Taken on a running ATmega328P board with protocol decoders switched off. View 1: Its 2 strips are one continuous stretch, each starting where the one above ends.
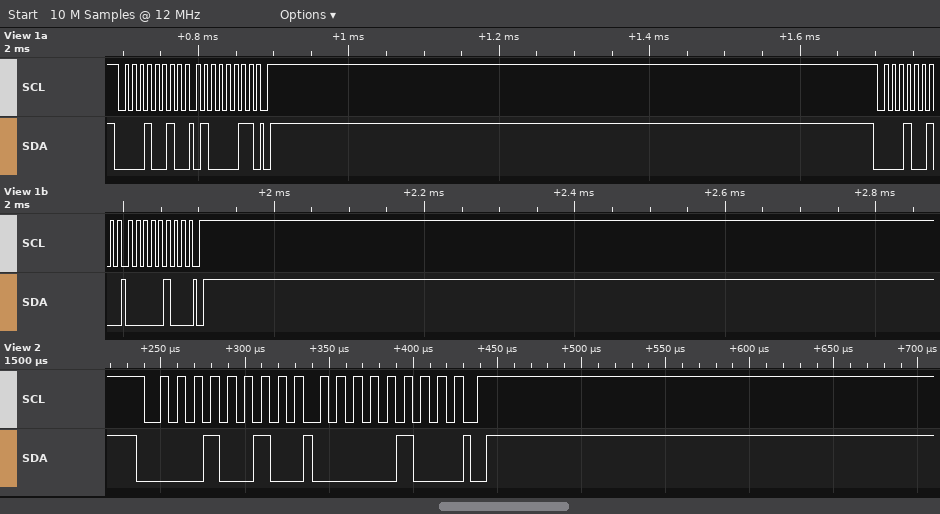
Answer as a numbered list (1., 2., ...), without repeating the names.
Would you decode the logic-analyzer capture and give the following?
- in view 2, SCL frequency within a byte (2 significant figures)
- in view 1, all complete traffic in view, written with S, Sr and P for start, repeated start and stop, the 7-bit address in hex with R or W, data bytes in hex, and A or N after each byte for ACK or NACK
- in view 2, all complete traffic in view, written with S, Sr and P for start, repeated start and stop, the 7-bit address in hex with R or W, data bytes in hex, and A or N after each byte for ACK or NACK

1. 100 kHz
2. S 09W A 43 A P S 09W A 04 A P
3. S 09W A 04 A P
